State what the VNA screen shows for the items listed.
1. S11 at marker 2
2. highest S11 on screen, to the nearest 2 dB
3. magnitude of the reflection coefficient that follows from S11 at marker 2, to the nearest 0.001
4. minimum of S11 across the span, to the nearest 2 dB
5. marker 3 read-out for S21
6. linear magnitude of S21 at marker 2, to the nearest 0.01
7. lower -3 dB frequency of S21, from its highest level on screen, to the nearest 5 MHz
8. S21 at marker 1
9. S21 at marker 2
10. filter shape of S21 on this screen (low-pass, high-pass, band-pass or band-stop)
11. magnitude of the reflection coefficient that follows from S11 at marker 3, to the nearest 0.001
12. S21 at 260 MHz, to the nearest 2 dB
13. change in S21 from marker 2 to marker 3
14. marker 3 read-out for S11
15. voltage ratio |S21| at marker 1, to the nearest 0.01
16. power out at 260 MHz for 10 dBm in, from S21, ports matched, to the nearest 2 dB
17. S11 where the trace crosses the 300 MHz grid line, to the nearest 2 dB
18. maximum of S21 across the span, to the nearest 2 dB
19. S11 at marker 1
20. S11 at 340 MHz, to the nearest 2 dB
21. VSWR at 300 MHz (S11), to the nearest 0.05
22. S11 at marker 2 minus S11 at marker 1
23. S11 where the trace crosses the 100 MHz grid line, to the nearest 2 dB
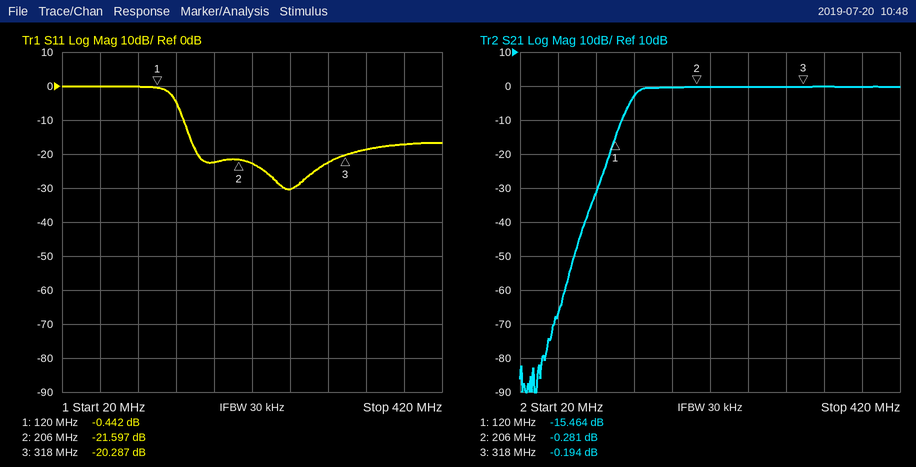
-21.597 dB
0 dB
0.083
-30 dB
-0.194 dB
0.97
140 MHz
-15.464 dB
-0.281 dB
high-pass
0.097
0 dB
0.087 dB
-20.287 dB
0.17
10 dBm
-22 dB
0 dB
-0.442 dB
-18 dB
1.15
-21.155 dB
0 dB
